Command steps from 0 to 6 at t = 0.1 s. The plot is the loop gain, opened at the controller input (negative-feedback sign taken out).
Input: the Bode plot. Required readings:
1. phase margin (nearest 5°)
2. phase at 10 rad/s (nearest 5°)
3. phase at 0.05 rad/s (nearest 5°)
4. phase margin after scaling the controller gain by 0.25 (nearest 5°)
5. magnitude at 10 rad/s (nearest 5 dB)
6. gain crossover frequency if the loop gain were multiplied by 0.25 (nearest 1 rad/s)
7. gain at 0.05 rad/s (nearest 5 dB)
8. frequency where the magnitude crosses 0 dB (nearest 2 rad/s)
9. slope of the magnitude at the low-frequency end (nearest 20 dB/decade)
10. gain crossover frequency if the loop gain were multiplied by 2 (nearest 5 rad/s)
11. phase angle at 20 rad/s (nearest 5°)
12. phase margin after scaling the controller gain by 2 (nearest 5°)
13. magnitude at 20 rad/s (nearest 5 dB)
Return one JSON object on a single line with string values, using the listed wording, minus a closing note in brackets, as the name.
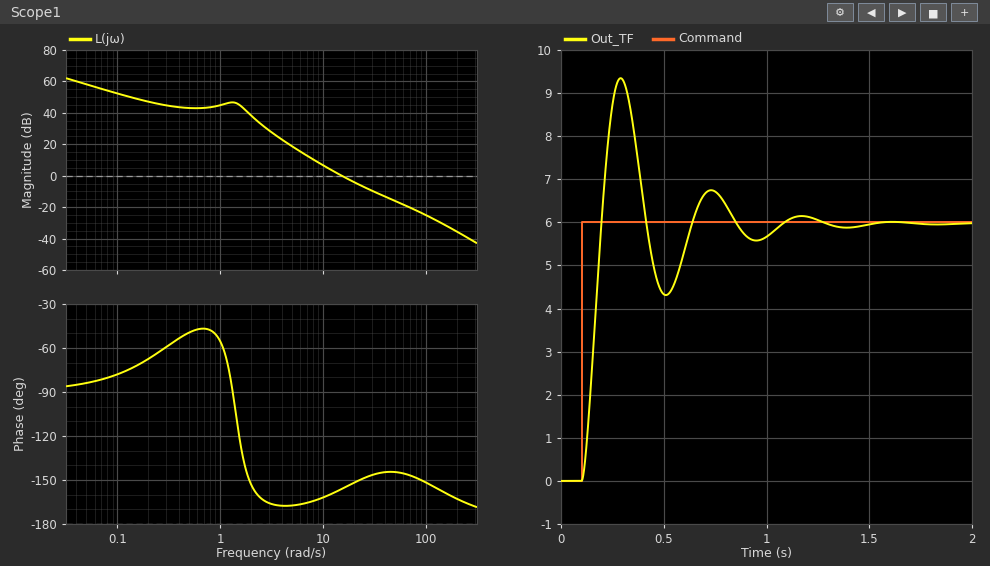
{"phase margin": "25°", "phase at 10 rad/s": "-160°", "phase at 0.05 rad/s": "-85°", "phase margin after scaling the controller gain by 0.25": "15°", "magnitude at 10 rad/s": "5 dB", "gain crossover frequency if the loop gain were multiplied by 0.25": "7 rad/s", "gain at 0.05 rad/s": "60 dB", "frequency where the magnitude crosses 0 dB": "16 rad/s", "slope of the magnitude at the low-frequency end": "-20 dB/decade", "gain crossover frequency if the loop gain were multiplied by 2": "25 rad/s", "phase angle at 20 rad/s": "-150°", "phase margin after scaling the controller gain by 2": "30°", "magnitude at 20 rad/s": "-5 dB"}
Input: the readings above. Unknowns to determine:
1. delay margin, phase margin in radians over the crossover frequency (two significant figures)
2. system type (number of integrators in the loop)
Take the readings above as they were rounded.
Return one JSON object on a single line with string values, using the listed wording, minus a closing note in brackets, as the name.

{"delay margin, phase margin in radians over the crossover frequency": "0.027 s", "system type": "1"}
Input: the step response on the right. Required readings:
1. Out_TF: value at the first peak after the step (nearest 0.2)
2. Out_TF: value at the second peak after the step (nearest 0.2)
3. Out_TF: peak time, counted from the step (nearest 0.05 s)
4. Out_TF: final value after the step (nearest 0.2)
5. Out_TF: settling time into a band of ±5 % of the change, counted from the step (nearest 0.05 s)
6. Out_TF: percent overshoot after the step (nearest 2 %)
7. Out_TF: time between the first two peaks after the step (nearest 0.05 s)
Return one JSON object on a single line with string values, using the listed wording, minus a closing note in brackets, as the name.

{"Out_TF: value at the first peak after the step": "9.4", "Out_TF: value at the second peak after the step": "6.8", "Out_TF: peak time, counted from the step": "0.20 s", "Out_TF: final value after the step": "6.0", "Out_TF: settling time into a band of ±5 % of the change, counted from the step": "0.90 s", "Out_TF: percent overshoot after the step": "56 %", "Out_TF: time between the first two peaks after the step": "0.45 s"}
